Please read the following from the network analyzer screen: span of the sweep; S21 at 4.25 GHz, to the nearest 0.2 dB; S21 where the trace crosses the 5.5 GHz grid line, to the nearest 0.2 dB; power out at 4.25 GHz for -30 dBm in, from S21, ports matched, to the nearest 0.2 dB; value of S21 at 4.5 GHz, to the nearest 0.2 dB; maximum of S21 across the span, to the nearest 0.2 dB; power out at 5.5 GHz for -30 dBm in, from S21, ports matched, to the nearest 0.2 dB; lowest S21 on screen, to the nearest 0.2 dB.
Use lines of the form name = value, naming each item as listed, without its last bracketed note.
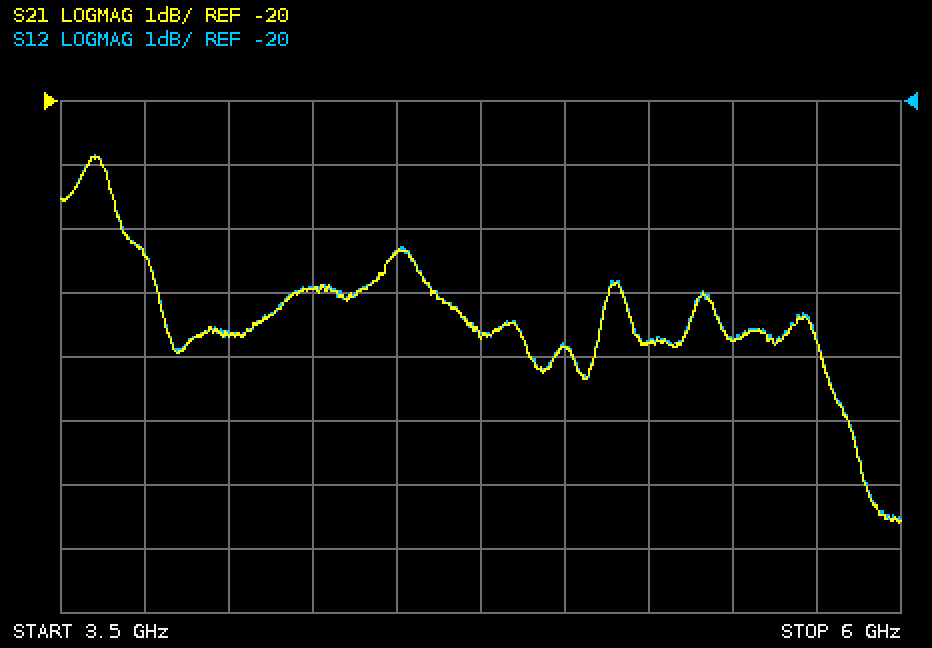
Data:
span of the sweep = 2.5 GHz
S21 at 4.25 GHz, to the nearest 0.2 dB = -23.0 dB
S21 where the trace crosses the 5.5 GHz grid line, to the nearest 0.2 dB = -23.8 dB
power out at 4.25 GHz for -30 dBm in, from S21, ports matched, to the nearest 0.2 dB = -53.0 dBm
value of S21 at 4.5 GHz, to the nearest 0.2 dB = -22.4 dB
maximum of S21 across the span, to the nearest 0.2 dB = -20.8 dB
power out at 5.5 GHz for -30 dBm in, from S21, ports matched, to the nearest 0.2 dB = -53.8 dBm
lowest S21 on screen, to the nearest 0.2 dB = -26.6 dB
